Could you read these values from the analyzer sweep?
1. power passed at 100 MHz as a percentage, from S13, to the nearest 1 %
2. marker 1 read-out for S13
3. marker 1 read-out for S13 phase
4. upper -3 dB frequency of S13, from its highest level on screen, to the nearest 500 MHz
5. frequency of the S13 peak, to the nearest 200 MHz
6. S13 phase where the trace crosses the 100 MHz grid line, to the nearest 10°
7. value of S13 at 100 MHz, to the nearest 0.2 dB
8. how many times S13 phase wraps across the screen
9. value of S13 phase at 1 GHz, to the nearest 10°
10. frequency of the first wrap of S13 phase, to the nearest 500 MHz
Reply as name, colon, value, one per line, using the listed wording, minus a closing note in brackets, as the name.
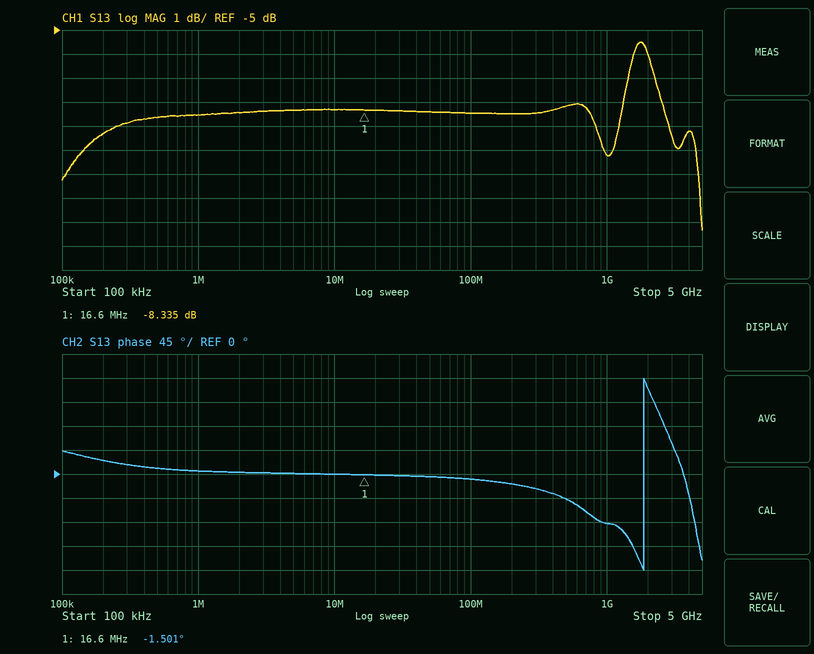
power passed at 100 MHz as a percentage, from S13, to the nearest 1 %: 14 %
marker 1 read-out for S13: -8.335 dB
marker 1 read-out for S13 phase: -1.501°
upper -3 dB frequency of S13, from its highest level on screen, to the nearest 500 MHz: 2.5 GHz
frequency of the S13 peak, to the nearest 200 MHz: 1.8 GHz
S13 phase where the trace crosses the 100 MHz grid line, to the nearest 10°: -10°
value of S13 at 100 MHz, to the nearest 0.2 dB: -8.4 dB
how many times S13 phase wraps across the screen: 1
value of S13 phase at 1 GHz, to the nearest 10°: -90°
frequency of the first wrap of S13 phase, to the nearest 500 MHz: 2.0 GHz
